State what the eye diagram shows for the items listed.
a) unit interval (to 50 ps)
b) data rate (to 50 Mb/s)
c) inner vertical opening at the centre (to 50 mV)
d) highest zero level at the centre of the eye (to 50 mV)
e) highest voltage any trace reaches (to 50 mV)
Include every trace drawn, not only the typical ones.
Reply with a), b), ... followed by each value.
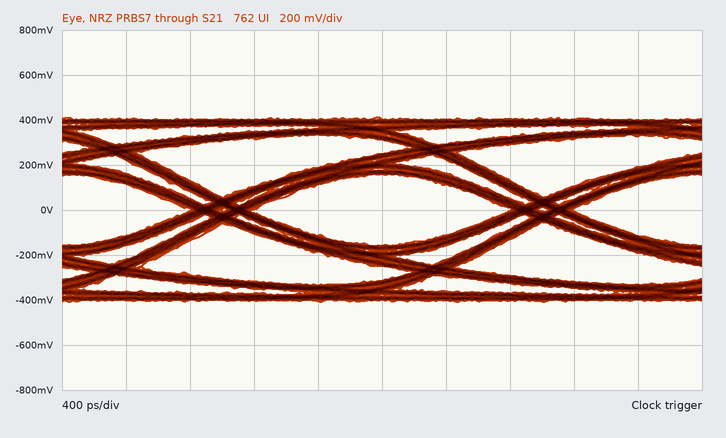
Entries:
a) 2.00 ns
b) 500 Mb/s
c) 300 mV
d) -150 mV
e) 400 mV
